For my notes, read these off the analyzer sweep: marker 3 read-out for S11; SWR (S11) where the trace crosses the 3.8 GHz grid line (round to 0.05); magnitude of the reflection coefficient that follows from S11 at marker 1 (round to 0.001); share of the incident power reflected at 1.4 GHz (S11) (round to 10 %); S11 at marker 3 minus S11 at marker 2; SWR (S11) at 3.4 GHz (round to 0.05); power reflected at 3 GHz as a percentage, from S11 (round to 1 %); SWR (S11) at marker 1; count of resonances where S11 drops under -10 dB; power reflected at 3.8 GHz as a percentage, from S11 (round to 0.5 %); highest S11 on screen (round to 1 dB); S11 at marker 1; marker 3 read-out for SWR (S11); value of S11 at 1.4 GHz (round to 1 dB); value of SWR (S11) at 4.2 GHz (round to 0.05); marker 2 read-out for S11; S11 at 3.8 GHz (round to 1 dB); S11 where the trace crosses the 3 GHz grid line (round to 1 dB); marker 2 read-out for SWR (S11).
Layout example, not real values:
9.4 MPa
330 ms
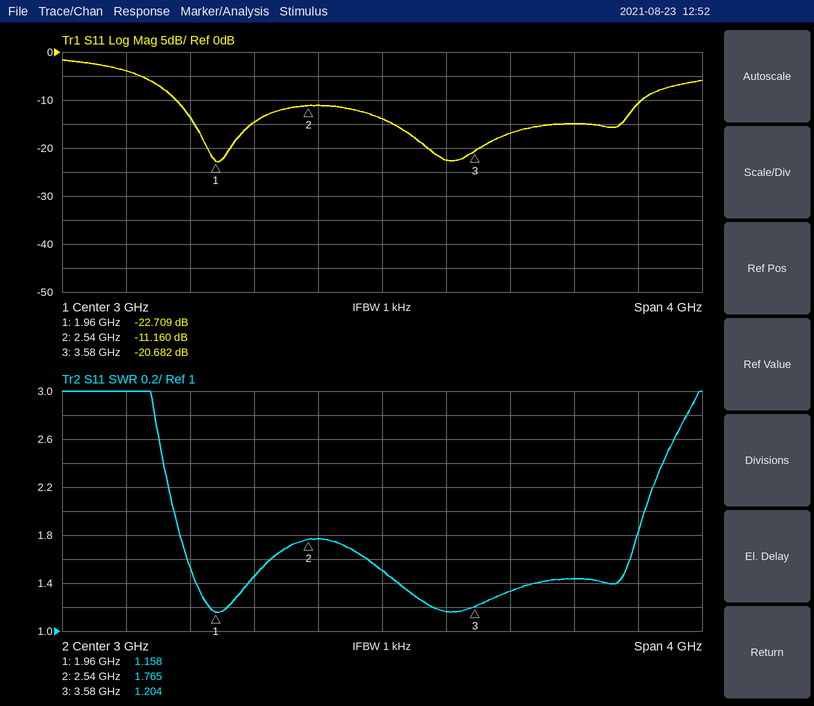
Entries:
-20.682 dB
1.35
0.073
40 %
-9.522 dB
1.15
4 %
1.158
2
2.0 %
-2 dB
-22.709 dB
1.204
-4 dB
1.45
-11.160 dB
-17 dB
-14 dB
1.765
